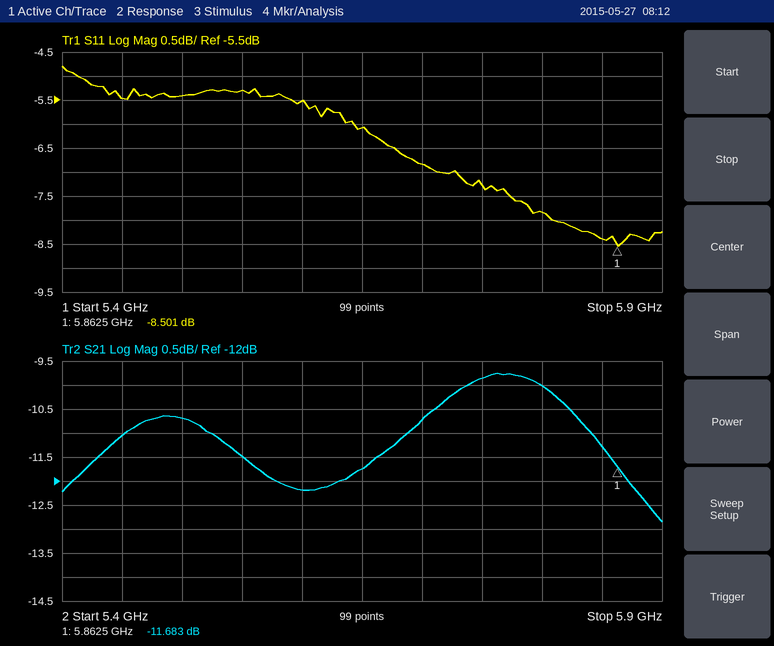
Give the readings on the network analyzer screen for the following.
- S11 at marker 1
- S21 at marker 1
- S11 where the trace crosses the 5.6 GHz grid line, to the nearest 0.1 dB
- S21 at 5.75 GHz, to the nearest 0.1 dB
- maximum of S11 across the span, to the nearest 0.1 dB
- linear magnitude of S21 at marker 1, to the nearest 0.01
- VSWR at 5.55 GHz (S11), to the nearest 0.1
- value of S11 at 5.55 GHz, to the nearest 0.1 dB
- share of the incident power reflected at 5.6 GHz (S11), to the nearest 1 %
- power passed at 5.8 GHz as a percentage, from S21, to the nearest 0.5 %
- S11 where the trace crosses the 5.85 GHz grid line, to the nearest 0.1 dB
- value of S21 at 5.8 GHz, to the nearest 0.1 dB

-8.501 dB
-11.683 dB
-5.5 dB
-9.9 dB
-4.8 dB
0.26
3.4
-5.3 dB
28 %
10.0 %
-8.4 dB
-10.0 dB
